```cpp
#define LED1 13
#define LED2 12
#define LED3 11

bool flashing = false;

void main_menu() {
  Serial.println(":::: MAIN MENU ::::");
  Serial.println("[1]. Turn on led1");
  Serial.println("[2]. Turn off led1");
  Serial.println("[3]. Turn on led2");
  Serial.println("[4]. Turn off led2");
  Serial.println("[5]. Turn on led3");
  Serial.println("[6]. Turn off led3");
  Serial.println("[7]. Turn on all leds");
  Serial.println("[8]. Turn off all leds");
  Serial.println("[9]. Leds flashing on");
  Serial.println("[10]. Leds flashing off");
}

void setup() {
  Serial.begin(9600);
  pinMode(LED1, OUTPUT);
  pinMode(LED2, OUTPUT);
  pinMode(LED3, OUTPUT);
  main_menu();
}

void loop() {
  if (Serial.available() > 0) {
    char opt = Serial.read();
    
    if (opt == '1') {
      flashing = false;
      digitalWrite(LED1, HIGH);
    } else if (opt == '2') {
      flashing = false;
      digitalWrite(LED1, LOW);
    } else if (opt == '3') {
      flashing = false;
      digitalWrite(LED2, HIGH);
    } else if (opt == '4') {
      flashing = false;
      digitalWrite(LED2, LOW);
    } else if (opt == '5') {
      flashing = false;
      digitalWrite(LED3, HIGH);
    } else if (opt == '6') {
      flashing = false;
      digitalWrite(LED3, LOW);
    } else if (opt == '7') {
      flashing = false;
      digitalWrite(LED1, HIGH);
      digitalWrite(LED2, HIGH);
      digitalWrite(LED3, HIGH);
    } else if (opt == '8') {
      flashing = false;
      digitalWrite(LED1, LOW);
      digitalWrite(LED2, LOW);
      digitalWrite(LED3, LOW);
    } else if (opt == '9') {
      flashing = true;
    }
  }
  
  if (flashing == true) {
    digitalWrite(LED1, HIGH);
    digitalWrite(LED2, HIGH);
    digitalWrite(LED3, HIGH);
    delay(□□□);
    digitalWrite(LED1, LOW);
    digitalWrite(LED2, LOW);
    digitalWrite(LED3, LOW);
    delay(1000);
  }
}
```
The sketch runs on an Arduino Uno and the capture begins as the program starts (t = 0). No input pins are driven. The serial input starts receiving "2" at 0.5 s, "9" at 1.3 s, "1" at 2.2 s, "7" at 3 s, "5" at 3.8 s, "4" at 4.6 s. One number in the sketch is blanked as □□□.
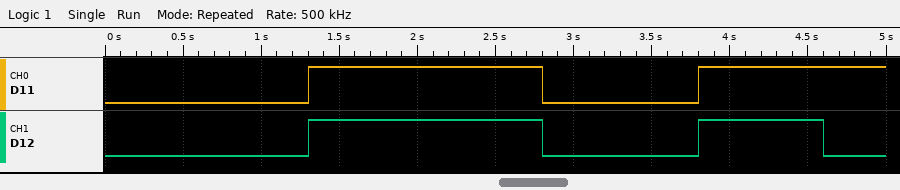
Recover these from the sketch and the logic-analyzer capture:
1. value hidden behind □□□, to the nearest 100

1500
